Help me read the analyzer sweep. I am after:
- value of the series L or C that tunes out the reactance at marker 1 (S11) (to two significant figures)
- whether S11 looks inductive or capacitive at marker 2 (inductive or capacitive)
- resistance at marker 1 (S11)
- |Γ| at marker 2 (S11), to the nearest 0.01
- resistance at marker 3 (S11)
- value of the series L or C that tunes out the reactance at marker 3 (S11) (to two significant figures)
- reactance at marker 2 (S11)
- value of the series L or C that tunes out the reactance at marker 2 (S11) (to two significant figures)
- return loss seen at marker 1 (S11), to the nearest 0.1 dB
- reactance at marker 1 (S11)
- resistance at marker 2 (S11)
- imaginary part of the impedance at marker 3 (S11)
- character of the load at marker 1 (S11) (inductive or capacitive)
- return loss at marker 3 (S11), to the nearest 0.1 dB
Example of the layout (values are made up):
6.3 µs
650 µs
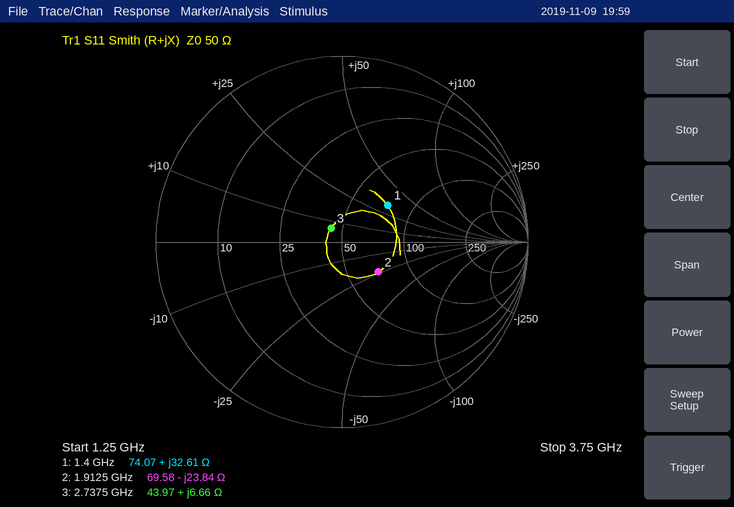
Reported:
3.5 pF
capacitive
74.07 Ω
0.25
43.97 Ω
8.7 pF
-23.84 Ω
2.0 nH
10.0 dB
+32.61 Ω
69.58 Ω
+6.66 Ω
inductive
20.4 dB
